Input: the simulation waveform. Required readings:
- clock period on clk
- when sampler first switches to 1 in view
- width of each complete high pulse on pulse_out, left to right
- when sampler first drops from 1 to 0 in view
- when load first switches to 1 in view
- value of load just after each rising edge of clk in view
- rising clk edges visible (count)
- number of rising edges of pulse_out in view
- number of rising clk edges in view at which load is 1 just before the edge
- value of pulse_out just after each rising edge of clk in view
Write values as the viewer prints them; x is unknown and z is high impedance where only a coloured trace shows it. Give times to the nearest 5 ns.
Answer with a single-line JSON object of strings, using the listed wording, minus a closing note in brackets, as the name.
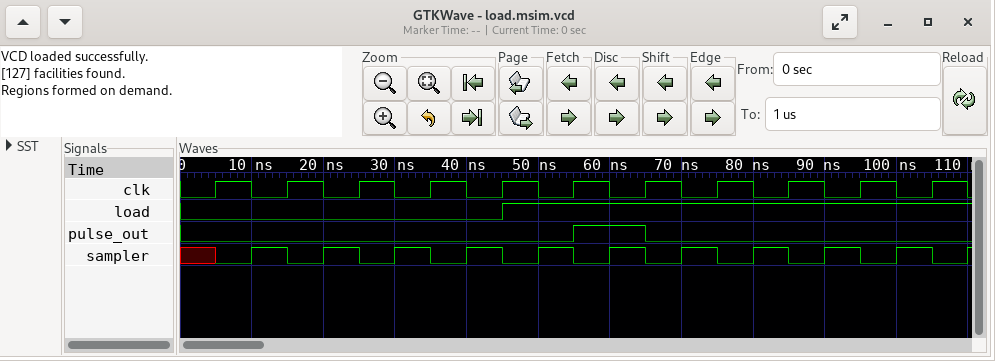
{"clock period on clk": "10 ns", "when sampler first switches to 1 in view": "10 ns", "width of each complete high pulse on pulse_out, left to right": "10 ns", "when sampler first drops from 1 to 0 in view": "15 ns", "when load first switches to 1 in view": "45 ns", "value of load just after each rising edge of clk in view": "0 0 0 0 1 1 1 1 1 1 1", "rising clk edges visible": "11", "number of rising edges of pulse_out in view": "1", "number of rising clk edges in view at which load is 1 just before the edge": "6", "value of pulse_out just after each rising edge of clk in view": "0 0 0 0 0 1 0 0 0 0 0"}
